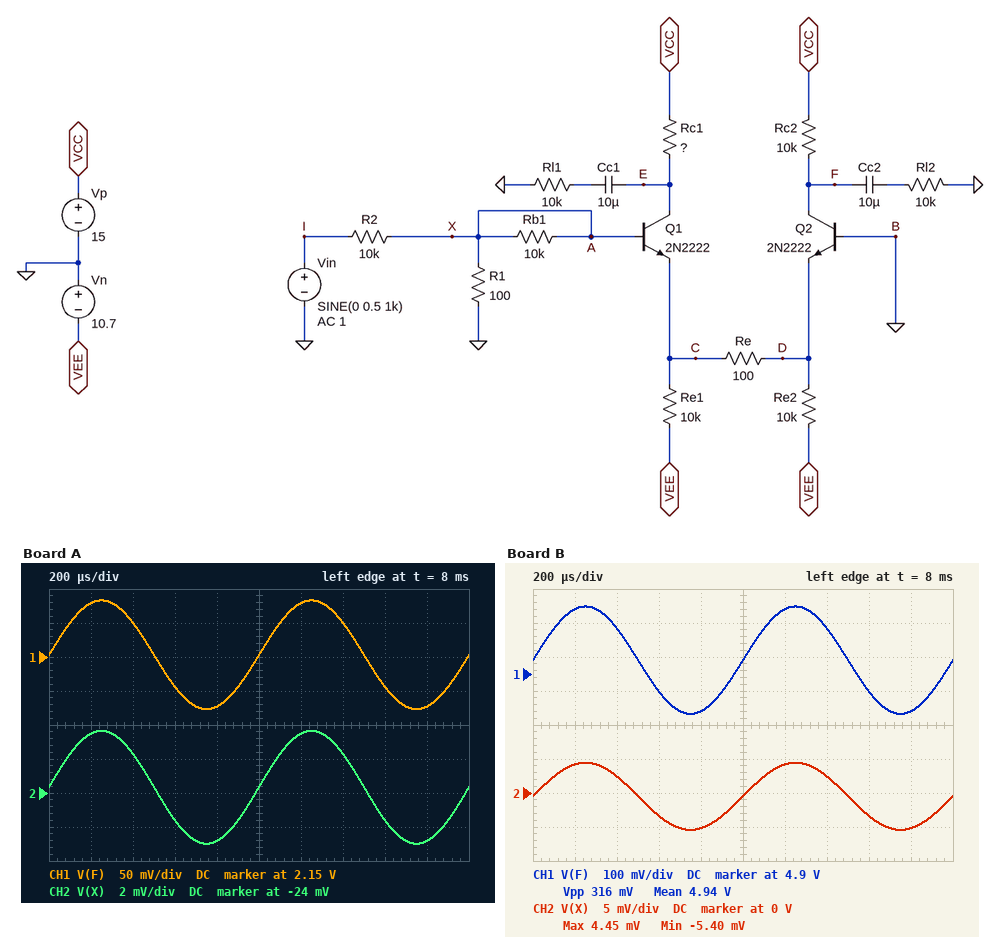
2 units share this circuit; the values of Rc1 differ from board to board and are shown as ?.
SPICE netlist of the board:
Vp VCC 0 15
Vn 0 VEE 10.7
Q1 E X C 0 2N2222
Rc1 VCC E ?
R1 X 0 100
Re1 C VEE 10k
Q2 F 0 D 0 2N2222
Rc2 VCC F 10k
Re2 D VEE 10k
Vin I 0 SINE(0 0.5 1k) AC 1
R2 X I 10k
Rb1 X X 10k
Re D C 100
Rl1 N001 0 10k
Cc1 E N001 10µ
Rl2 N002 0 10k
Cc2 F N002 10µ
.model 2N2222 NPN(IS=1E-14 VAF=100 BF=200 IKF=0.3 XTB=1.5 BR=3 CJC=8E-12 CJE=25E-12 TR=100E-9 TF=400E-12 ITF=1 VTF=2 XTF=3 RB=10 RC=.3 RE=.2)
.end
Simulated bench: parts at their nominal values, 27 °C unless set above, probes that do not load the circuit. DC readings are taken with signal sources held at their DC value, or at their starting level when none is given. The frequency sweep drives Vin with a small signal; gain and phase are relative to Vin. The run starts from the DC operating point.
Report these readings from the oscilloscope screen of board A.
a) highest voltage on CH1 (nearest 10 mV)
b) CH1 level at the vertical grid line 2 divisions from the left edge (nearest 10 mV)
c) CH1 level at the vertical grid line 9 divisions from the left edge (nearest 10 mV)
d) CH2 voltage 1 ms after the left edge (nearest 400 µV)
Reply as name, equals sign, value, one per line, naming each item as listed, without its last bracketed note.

highest voltage on CH1 = 2.23 V
CH1 level at the vertical grid line 2 divisions from the left edge = 2.20 V
CH1 level at the vertical grid line 9 divisions from the left edge = 2.08 V
CH2 voltage 1 ms after the left edge = -23.6 mV
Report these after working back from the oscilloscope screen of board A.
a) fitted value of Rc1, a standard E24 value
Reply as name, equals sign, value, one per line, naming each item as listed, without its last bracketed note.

fitted value of Rc1, a standard E24 value = 33 kΩ
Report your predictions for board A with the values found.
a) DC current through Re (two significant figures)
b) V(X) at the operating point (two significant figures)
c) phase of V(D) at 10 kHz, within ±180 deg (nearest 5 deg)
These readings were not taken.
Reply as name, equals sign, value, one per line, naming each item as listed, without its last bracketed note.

DC current through Re = 290 µA
V(X) at the operating point = -24 mV
phase of V(D) at 10 kHz, within ±180 deg = 0 deg
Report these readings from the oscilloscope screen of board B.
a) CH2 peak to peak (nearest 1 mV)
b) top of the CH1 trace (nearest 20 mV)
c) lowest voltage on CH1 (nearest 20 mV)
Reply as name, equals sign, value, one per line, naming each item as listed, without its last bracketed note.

CH2 peak to peak = 10 mV
top of the CH1 trace = 5.10 V
lowest voltage on CH1 = 4.78 V
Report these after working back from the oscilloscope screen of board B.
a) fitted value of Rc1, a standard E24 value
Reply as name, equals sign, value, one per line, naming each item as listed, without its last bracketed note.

fitted value of Rc1, a standard E24 value = 12 kΩ
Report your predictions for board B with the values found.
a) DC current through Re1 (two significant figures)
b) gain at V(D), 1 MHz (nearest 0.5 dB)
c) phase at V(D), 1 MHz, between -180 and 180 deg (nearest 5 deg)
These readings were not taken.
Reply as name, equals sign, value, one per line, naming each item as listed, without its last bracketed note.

DC current through Re1 = 1.0 mA
gain at V(D), 1 MHz = -55.5 dB
phase at V(D), 1 MHz, between -180 and 180 deg = -5 deg
